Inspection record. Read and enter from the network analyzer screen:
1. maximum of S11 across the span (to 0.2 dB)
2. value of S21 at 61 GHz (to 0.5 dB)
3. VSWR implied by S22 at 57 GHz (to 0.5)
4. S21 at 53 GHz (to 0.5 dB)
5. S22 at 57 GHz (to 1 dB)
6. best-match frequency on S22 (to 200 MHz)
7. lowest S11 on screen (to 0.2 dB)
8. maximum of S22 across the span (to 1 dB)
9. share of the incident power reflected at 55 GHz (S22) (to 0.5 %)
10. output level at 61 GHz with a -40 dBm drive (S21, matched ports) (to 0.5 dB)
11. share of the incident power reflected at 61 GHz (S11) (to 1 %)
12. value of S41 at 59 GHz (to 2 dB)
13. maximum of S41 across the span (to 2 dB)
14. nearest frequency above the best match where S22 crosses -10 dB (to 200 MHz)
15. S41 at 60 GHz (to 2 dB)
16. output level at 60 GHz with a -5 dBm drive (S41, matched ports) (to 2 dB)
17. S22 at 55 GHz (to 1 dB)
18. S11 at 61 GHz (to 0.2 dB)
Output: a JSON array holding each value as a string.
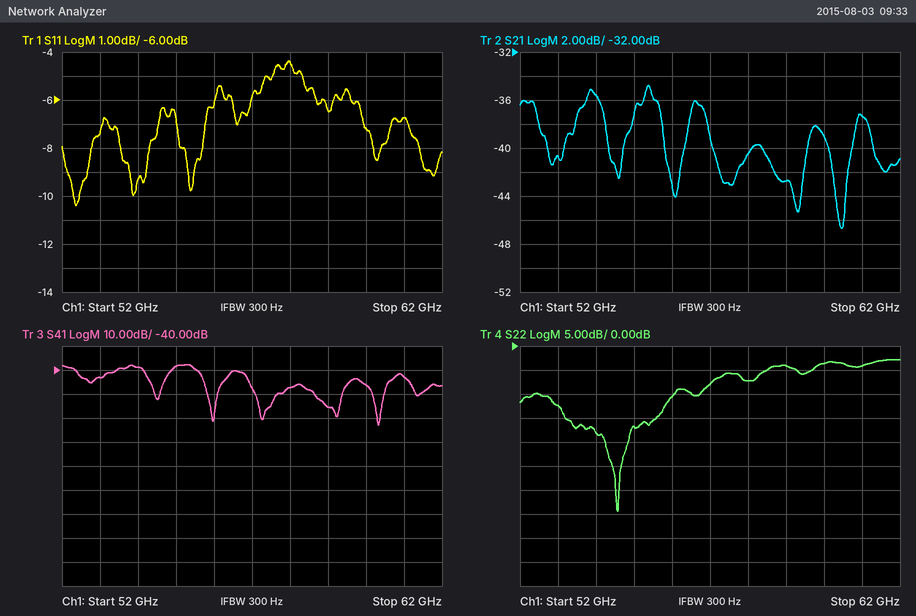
["-4.4 dB", "-37.5 dB", "2.5", "-40.5 dB", "-8 dB", "54.6 GHz", "-10.4 dB", "-3 dB", "2.0 %", "-77.5 dBm", "21 %", "-56 dB", "-38 dB", "56.0 GHz", "-46 dB", "-52 dBm", "-17 dB", "-6.8 dB"]
